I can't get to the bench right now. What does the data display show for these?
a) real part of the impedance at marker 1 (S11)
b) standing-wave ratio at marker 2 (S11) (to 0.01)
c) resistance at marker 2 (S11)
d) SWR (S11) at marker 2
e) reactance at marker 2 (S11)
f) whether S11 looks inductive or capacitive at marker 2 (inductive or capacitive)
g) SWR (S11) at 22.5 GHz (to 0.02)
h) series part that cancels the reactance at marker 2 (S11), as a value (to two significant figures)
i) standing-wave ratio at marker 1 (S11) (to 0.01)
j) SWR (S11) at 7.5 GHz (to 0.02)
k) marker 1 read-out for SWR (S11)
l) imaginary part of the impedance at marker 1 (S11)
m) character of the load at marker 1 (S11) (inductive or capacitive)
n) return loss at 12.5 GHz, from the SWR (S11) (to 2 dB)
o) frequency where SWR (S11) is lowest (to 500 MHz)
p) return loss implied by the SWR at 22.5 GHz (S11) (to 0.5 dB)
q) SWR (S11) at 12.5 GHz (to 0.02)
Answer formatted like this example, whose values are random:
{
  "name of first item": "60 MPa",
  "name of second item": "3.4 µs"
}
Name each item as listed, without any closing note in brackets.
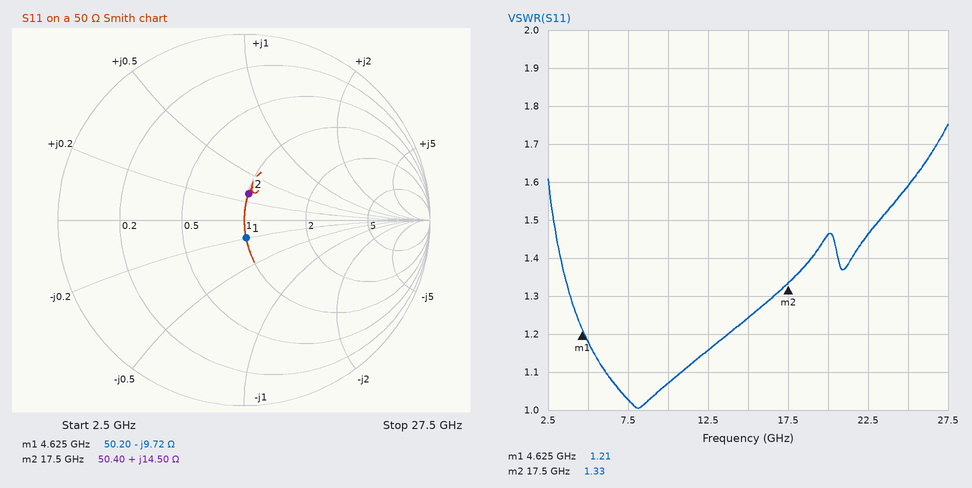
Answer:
{
  "real part of the impedance at marker 1": "50.20 Ω",
  "standing-wave ratio at marker 2 (S11)": "1.33",
  "resistance at marker 2": "50.40 Ω",
  "SWR (S11) at marker 2": "1.33",
  "reactance at marker 2": "+14.50 Ω",
  "whether S11 looks inductive or capacitive at marker 2": "inductive",
  "SWR (S11) at 22.5 GHz": "1.46",
  "series part that cancels the reactance at marker 2 (S11), as a value": "630 fF",
  "standing-wave ratio at marker 1 (S11)": "1.21",
  "SWR (S11) at 7.5 GHz": "1.02",
  "marker 1 read-out for SWR": "1.21",
  "imaginary part of the impedance at marker 1": "-9.72 Ω",
  "character of the load at marker 1 (S11)": "capacitive",
  "return loss at 12.5 GHz, from the SWR (S11)": "22 dB",
  "frequency where SWR (S11) is lowest": "8.0 GHz",
  "return loss implied by the SWR at 22.5 GHz (S11)": "14.5 dB",
  "SWR (S11) at 12.5 GHz": "1.16"
}
